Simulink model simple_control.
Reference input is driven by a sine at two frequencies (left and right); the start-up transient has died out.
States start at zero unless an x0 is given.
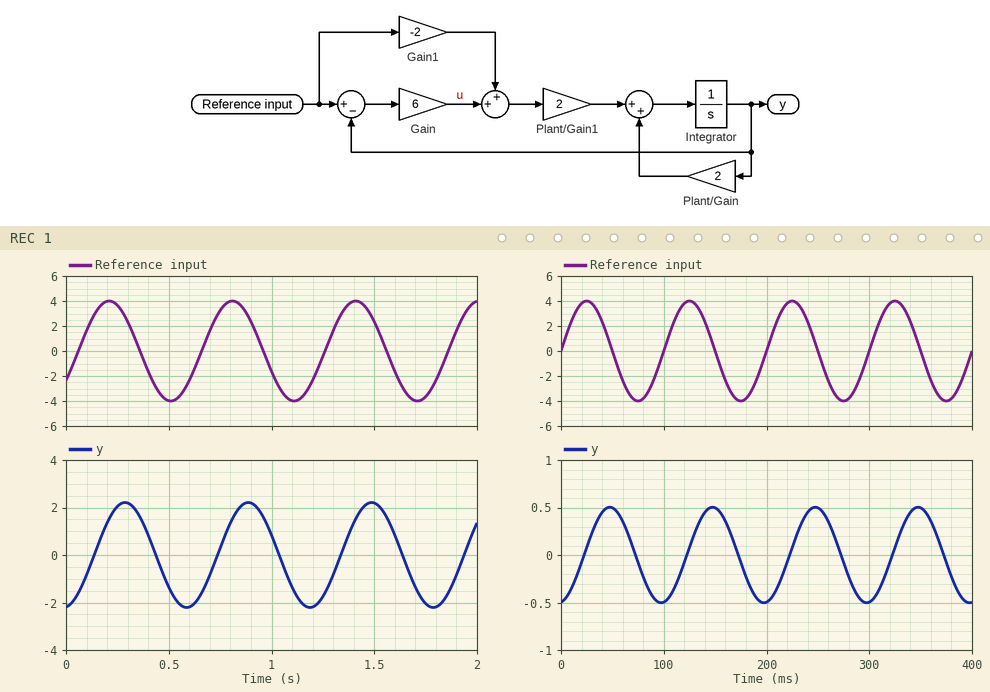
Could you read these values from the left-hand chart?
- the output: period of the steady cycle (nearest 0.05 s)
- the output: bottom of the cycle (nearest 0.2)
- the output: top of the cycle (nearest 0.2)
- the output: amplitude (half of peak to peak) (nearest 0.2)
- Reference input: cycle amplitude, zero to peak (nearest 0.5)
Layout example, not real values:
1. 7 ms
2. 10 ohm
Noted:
1. 0.60 s
2. -2.2
3. 2.2
4. 2.2
5. 4.0
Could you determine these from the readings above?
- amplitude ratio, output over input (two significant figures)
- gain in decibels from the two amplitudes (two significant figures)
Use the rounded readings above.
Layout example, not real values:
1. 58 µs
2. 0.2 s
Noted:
1. 0.55
2. -5.2 dB
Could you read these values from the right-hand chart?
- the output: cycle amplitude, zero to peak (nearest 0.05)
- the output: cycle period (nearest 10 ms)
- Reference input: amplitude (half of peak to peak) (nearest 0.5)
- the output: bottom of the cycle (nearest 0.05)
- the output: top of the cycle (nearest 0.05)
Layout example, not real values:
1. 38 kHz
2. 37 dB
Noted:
1. 0.50
2. 100 ms
3. 4.0
4. -0.50
5. 0.50
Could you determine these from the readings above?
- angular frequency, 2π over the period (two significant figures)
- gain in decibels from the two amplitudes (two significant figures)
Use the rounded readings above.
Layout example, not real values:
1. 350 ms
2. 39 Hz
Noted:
1. 0.063 rad/ms
2. -18 dB
